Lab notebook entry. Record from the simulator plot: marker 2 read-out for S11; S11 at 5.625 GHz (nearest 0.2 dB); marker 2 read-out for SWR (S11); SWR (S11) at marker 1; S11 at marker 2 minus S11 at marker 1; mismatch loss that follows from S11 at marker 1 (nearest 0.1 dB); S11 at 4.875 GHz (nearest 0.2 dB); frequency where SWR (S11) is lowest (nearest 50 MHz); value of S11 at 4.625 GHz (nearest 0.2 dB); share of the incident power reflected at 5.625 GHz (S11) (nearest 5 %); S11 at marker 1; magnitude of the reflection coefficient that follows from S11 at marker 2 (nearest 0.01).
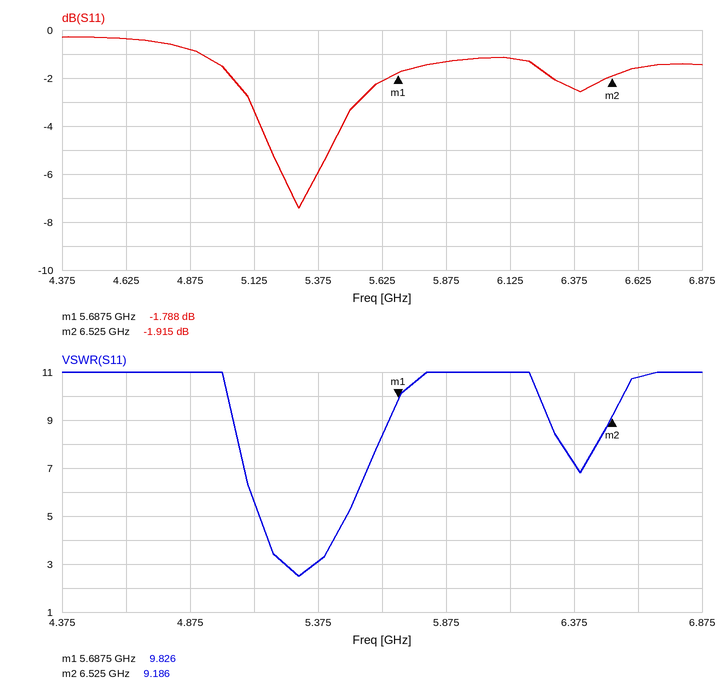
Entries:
-1.915 dB
-2.2 dB
9.186
9.826
-0.127 dB
4.7 dB
-0.8 dB
5.30 GHz
-0.4 dB
60 %
-1.788 dB
0.80
